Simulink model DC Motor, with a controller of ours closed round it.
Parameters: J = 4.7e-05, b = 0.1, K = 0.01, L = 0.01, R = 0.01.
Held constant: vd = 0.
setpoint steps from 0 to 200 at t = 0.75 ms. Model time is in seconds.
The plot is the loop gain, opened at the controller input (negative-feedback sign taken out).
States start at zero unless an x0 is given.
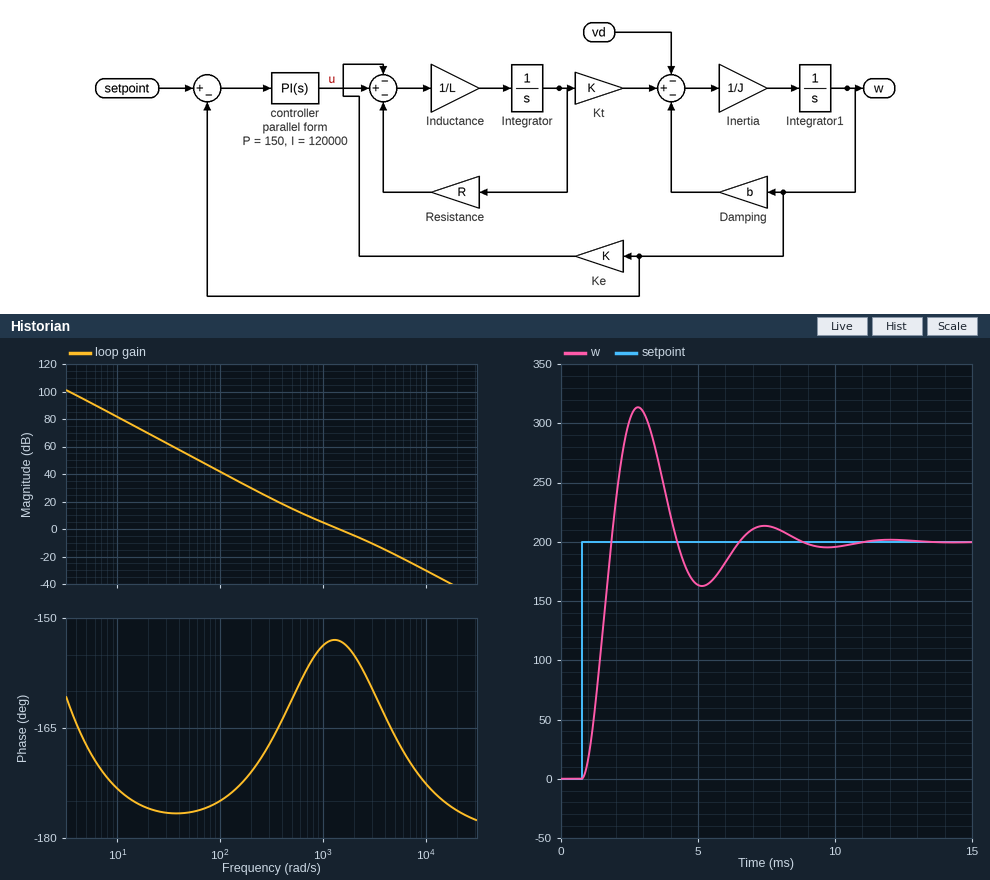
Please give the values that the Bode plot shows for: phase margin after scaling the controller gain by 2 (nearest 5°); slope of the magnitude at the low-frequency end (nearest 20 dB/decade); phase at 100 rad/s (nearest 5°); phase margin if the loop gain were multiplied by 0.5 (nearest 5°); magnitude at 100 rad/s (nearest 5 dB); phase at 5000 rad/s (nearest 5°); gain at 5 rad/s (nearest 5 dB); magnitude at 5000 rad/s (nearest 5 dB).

25°
-40 dB/decade
-175°
25°
40 dB
-165°
95 dB
-20 dB
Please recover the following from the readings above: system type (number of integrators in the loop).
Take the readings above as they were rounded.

2
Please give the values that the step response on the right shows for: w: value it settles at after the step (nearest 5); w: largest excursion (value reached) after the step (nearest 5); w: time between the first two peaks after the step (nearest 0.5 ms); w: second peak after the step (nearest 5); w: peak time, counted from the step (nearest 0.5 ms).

200
315
4.5 ms
215
2.0 ms
